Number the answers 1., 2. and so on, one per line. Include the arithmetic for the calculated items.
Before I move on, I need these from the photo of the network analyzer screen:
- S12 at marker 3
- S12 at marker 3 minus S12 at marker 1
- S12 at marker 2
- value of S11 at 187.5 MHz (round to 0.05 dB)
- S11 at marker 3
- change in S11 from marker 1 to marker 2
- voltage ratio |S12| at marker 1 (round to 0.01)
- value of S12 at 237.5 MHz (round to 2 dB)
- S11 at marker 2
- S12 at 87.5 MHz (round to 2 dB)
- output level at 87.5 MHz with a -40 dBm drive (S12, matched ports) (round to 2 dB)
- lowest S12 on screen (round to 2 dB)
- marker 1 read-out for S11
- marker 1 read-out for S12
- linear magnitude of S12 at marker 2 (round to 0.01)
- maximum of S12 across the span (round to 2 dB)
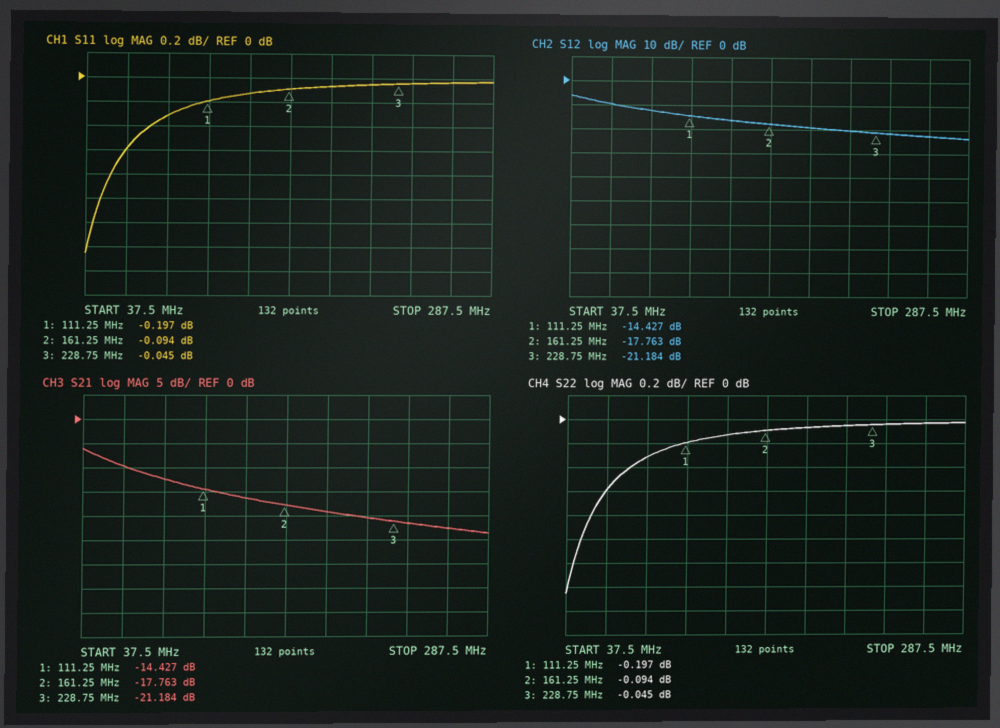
1. -21.184 dB
2. -21.184 − (-14.427) = -6.757 dB
3. -17.763 dB
4. -0.05 dB
5. -0.045 dB
6. -0.094 − (-0.197) = 0.103 dB
7. 10^(-14.427/20) ≈ 0.19
8. -22 dB
9. -0.094 dB
10. -12 dB
11. -40 dBm + (-12 dB) = -52 dBm
12. -24 dB
13. -0.197 dB
14. -14.427 dB
15. 10^(-17.763/20) ≈ 0.13
16. -6 dB
